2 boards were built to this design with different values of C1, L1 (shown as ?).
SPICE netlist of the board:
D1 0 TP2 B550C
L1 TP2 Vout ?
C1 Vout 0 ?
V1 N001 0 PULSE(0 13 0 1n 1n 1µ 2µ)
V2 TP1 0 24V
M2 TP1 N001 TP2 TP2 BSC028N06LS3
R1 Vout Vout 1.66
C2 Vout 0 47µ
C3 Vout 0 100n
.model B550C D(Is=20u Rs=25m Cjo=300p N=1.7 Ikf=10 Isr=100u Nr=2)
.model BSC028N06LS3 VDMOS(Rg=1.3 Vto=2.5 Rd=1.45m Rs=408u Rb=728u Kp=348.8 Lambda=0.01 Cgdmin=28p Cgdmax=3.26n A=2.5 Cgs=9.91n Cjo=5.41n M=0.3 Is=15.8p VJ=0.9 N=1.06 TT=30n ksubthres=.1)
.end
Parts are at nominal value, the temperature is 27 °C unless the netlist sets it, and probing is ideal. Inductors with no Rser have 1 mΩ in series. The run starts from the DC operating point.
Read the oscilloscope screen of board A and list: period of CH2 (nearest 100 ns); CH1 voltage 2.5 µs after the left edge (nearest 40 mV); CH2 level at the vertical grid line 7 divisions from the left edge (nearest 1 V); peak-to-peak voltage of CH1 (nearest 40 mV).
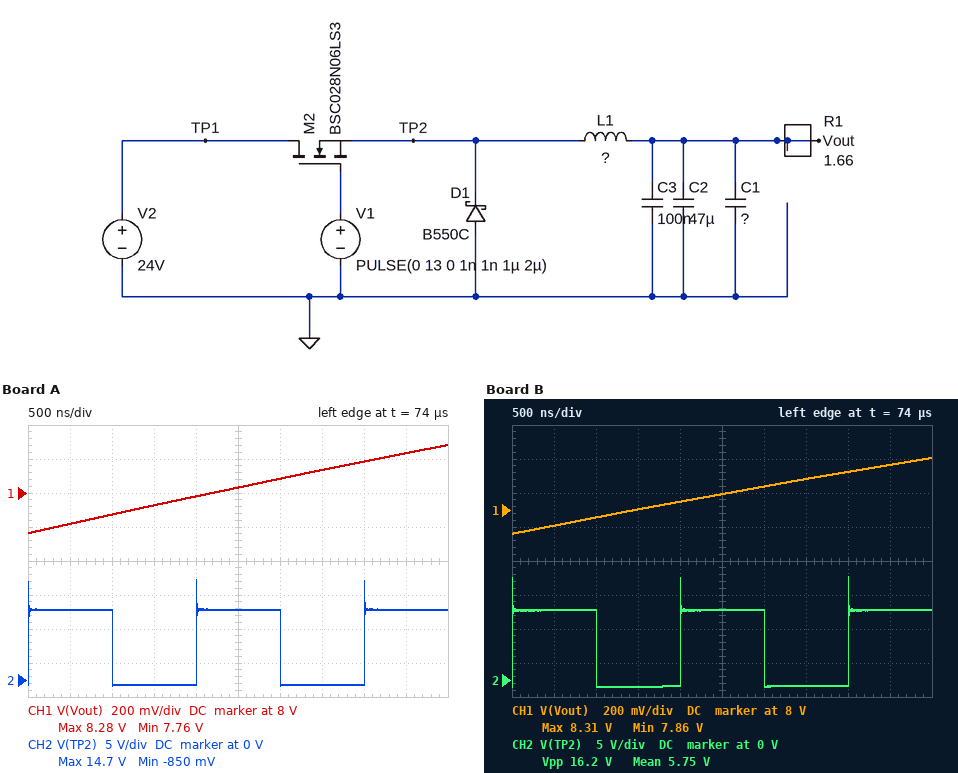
2.0 µs
8.04 V
-1 V
520 mV
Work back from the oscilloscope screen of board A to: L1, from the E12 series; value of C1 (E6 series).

18 µH
15 µF
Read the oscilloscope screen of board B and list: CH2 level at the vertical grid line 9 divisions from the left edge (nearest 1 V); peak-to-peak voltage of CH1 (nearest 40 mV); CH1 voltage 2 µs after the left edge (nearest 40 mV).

10 V
440 mV
8.04 V
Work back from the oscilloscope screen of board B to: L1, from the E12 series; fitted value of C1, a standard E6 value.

6.8 µH
100 µF
